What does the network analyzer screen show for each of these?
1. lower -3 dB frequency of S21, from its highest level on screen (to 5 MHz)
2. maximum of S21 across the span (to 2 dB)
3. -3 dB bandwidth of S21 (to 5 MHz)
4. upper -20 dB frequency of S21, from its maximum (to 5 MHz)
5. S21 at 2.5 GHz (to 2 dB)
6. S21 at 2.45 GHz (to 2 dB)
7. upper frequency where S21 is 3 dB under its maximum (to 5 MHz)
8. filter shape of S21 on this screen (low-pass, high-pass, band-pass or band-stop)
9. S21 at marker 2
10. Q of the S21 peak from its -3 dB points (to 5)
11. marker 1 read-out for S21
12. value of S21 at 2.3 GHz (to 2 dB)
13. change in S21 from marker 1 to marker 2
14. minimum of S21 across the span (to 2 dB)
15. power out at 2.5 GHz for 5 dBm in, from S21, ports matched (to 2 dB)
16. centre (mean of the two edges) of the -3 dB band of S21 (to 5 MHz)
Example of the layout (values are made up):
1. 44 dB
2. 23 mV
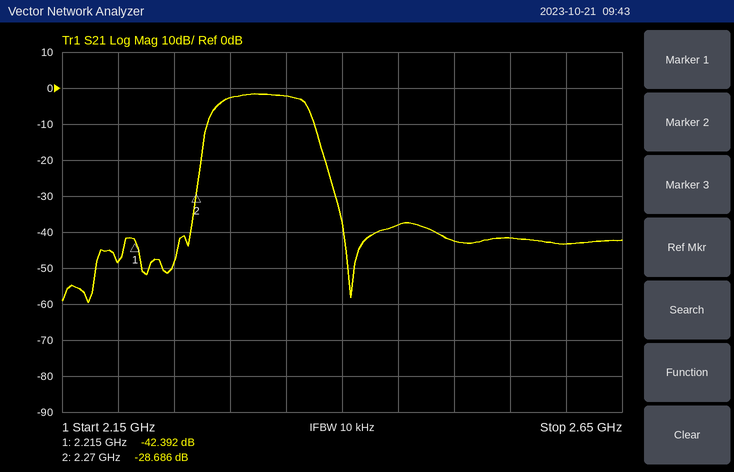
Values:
1. 2.290 GHz
2. -2 dB
3. 80 MHz
4. 2.385 GHz
5. -42 dB
6. -38 dB
7. 2.370 GHz
8. band-pass
9. -28.686 dB
10. 30
11. -42.392 dB
12. -2 dB
13. 13.706 dB
14. -60 dB
15. -38 dBm
16. 2.330 GHz
